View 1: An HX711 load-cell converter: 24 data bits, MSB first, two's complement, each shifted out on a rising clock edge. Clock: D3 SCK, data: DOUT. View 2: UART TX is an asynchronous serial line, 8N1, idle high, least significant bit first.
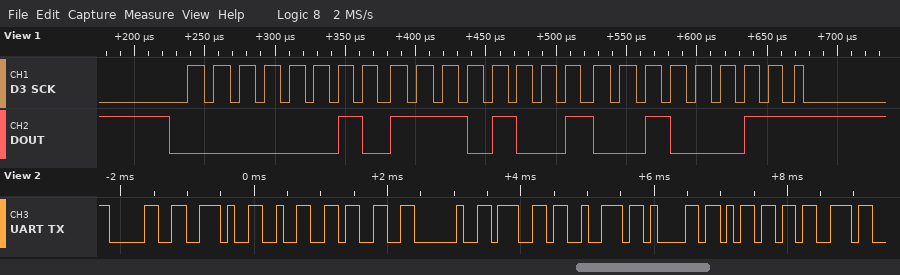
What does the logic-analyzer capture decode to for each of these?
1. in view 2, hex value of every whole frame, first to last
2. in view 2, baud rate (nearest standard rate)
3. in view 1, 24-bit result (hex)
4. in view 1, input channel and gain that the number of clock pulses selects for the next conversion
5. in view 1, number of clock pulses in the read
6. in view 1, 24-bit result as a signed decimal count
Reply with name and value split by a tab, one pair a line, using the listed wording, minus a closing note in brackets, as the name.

in view 2, hex value of every whole frame, first to last	0x30 0x2E 0x32 0x33 0x20 0x67 0x72 0x61 0x6D 0x73
in view 2, baud rate	9600 baud
in view 1, 24-bit result	0x02E923
in view 1, input channel and gain that the number of clock pulses selects for the next conversion	channel A, gain 128
in view 1, number of clock pulses in the read	25
in view 1, 24-bit result as a signed decimal count	190755
